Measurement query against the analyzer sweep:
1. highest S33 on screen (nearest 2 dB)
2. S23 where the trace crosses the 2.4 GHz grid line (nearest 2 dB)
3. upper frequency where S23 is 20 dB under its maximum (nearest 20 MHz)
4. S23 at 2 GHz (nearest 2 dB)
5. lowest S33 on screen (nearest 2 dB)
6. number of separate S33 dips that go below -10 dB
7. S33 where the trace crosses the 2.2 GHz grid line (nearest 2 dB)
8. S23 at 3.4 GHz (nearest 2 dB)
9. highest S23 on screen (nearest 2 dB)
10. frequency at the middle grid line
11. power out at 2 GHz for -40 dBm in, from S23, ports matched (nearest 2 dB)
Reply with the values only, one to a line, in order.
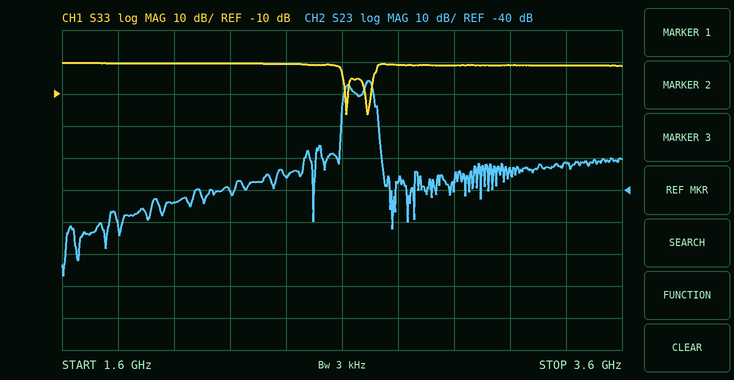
0 dB
-36 dB
2.74 GHz
-44 dB
-16 dB
2
0 dB
-32 dB
-6 dB
2.6 GHz
-84 dBm
